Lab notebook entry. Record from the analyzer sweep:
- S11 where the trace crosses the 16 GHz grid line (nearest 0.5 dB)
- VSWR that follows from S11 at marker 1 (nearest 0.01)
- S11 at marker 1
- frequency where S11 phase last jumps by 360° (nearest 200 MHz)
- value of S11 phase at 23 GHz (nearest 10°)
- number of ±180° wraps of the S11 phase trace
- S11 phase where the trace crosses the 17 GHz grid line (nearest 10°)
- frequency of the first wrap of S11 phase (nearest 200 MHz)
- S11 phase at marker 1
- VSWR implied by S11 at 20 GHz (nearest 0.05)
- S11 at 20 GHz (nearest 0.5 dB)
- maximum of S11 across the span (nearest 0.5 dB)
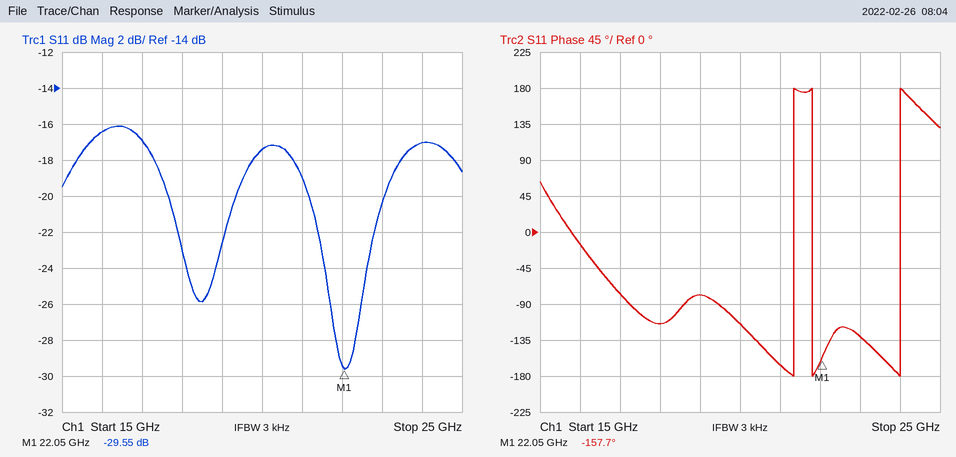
-16.5 dB
1.07
-29.55 dB
24.0 GHz
-130°
3
-80°
21.4 GHz
-157.7°
1.30
-17.5 dB
-16.0 dB
